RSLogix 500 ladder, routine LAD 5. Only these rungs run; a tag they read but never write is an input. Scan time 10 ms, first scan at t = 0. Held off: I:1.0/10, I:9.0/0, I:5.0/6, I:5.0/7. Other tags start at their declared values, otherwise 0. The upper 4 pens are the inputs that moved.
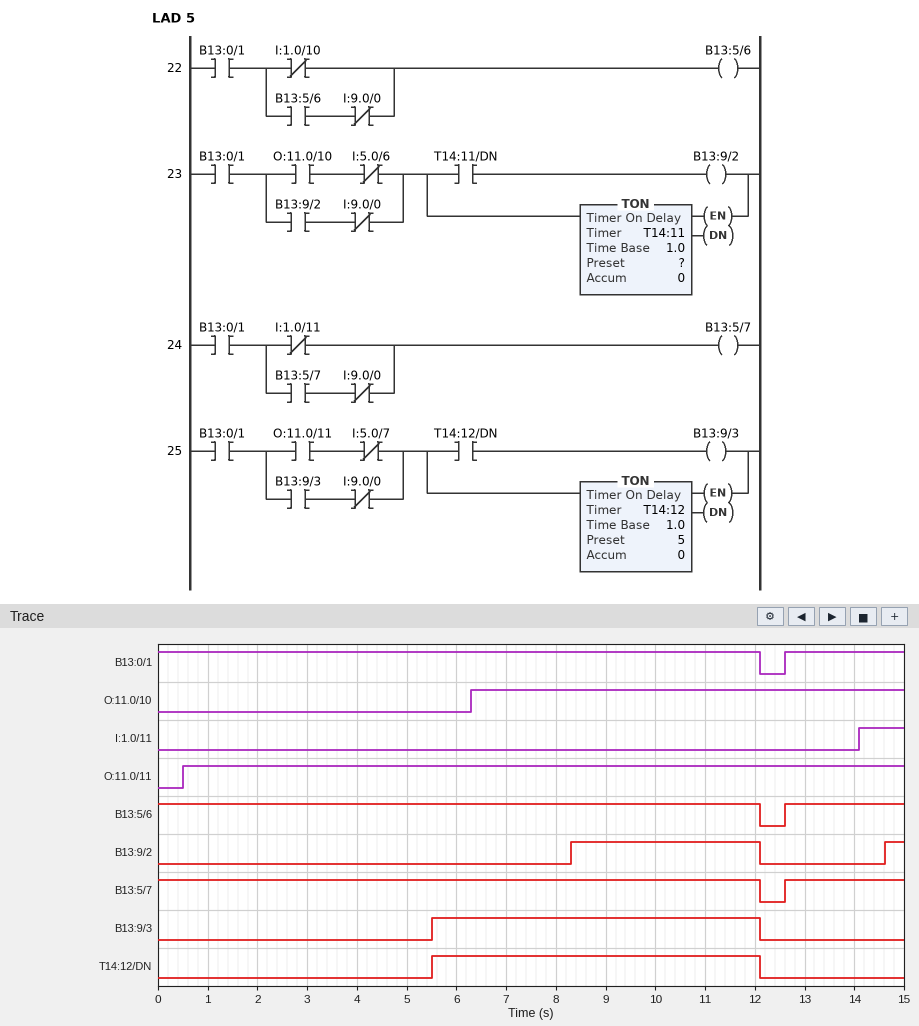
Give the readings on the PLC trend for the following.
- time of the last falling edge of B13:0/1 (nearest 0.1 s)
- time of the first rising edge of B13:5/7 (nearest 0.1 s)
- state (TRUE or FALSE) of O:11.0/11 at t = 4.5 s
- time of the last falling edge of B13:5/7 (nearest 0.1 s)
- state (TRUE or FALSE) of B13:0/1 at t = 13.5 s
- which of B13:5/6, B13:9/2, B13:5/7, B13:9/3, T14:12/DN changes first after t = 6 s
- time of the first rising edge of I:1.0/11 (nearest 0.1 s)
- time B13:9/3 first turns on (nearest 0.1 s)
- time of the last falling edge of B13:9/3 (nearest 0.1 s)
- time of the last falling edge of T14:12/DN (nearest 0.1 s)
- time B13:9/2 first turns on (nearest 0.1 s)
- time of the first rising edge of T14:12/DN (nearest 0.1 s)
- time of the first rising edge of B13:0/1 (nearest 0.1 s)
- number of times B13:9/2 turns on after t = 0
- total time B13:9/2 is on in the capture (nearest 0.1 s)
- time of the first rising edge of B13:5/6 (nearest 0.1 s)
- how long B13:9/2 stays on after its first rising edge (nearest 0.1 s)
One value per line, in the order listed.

12.1 s
12.6 s
TRUE
12.1 s
TRUE
B13:9/2
14.1 s
5.5 s
12.1 s
12.1 s
8.3 s
5.5 s
12.6 s
2
4.2 s
12.6 s
3.8 s
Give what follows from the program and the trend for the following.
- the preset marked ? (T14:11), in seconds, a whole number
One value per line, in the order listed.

2 s
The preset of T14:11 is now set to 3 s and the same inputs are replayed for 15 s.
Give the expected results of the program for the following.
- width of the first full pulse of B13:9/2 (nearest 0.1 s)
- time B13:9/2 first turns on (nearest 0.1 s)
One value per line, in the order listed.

2.8 s
9.3 s
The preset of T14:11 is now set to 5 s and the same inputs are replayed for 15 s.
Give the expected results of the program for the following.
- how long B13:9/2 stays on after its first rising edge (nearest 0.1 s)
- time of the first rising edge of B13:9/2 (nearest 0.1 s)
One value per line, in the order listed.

0.8 s
11.3 s
